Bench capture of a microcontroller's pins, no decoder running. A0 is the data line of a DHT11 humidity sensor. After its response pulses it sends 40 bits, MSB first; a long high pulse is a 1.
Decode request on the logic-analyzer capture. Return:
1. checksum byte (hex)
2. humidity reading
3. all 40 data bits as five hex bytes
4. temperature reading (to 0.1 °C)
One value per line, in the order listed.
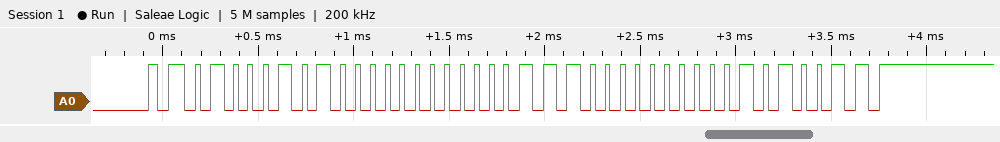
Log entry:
0x53
69 %
45 00 0E 00 53
14.0 °C
